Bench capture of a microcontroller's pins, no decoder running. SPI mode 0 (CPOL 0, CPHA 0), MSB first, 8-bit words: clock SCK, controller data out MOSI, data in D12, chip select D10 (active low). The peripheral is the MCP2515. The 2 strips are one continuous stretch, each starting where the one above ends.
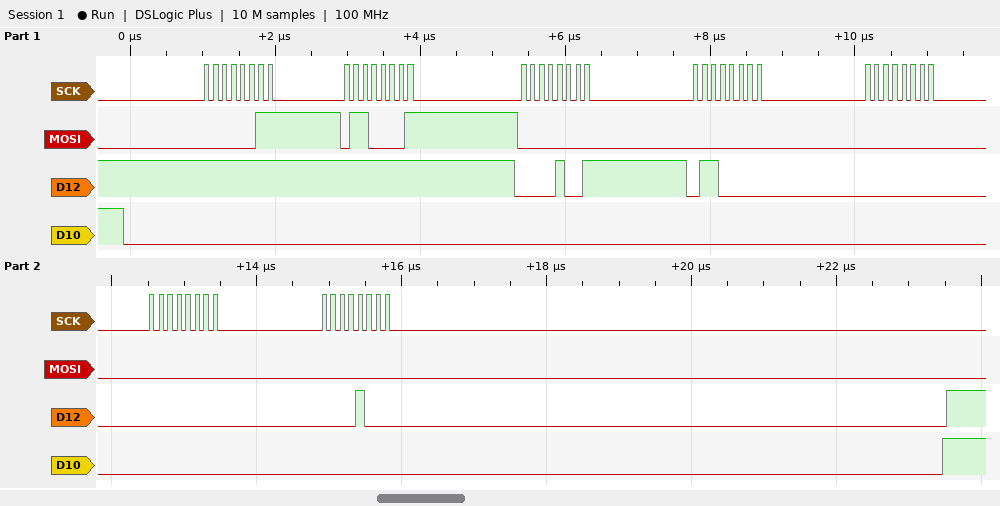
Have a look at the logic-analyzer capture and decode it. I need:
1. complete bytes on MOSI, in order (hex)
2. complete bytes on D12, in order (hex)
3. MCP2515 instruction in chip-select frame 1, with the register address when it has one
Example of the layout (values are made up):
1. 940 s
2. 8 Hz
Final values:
1. 0x03 0x61 0x00 0x00 0x00 0x00 0x00
2. 0xFF 0xFF 0x09 0x60 0x00 0x00 0x08
3. READ 0x61
